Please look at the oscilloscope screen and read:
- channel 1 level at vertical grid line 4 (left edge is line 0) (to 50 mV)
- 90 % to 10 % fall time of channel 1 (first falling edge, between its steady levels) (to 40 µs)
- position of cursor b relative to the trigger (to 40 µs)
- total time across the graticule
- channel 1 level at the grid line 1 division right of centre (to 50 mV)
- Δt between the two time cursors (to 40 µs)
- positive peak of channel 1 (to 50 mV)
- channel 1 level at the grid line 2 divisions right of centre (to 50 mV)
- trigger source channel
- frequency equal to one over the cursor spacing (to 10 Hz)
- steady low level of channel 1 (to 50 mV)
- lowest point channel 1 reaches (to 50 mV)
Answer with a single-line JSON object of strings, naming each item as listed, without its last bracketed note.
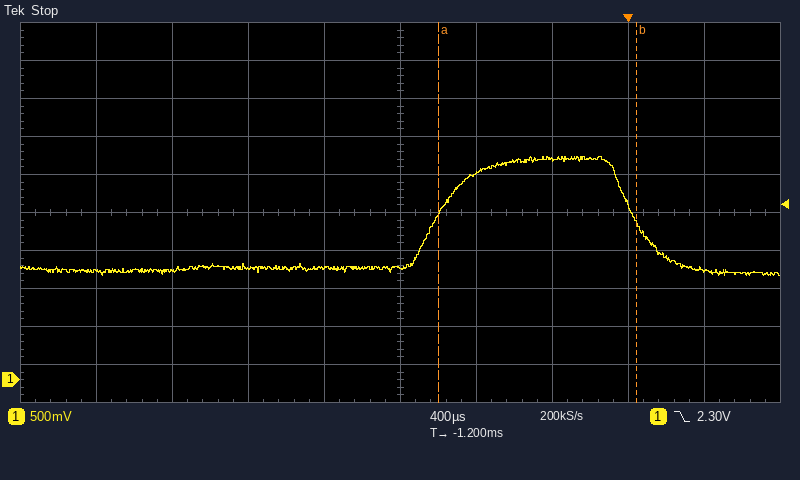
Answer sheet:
{"channel 1 level at vertical grid line 4 (left edge is line 0)": "1.45 V", "90 % to 10 % fall time of channel 1 (first falling edge, between its steady levels)": "280 µs", "position of cursor b relative to the trigger": "+40 µs", "total time across the graticule": "4 ms", "channel 1 level at the grid line 1 division right of centre": "2.70 V", "Δt between the two time cursors": "1.04 ms", "positive peak of channel 1": "2.95 V", "channel 1 level at the grid line 2 divisions right of centre": "2.90 V", "trigger source channel": "channel 1", "frequency equal to one over the cursor spacing": "960 Hz", "steady low level of channel 1": "1.45 V", "lowest point channel 1 reaches": "1.35 V"}
